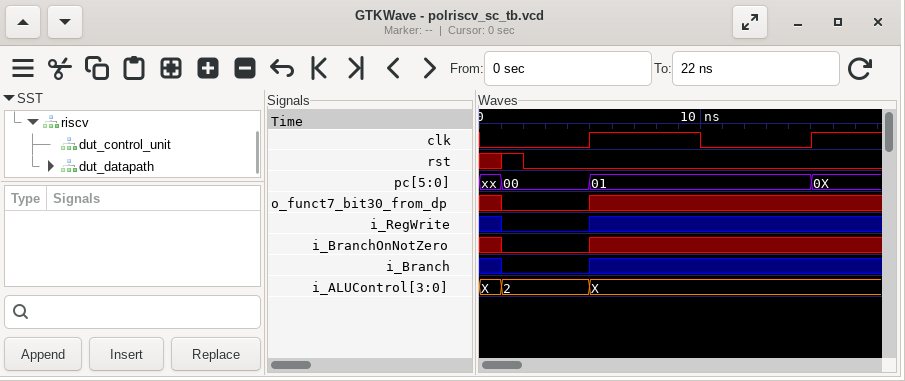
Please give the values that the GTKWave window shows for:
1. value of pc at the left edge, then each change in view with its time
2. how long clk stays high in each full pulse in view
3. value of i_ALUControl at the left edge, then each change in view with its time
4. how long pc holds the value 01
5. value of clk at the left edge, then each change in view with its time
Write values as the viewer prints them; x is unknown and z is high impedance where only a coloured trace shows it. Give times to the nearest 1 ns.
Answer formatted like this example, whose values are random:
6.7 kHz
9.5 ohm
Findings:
xx, 00 at 1 ns, 01 at 5 ns, 0X at 15 ns
5 ns
X, 2 at 1 ns, X at 5 ns
10 ns
0, 1 at 5 ns, 0 at 10 ns, 1 at 15 ns
